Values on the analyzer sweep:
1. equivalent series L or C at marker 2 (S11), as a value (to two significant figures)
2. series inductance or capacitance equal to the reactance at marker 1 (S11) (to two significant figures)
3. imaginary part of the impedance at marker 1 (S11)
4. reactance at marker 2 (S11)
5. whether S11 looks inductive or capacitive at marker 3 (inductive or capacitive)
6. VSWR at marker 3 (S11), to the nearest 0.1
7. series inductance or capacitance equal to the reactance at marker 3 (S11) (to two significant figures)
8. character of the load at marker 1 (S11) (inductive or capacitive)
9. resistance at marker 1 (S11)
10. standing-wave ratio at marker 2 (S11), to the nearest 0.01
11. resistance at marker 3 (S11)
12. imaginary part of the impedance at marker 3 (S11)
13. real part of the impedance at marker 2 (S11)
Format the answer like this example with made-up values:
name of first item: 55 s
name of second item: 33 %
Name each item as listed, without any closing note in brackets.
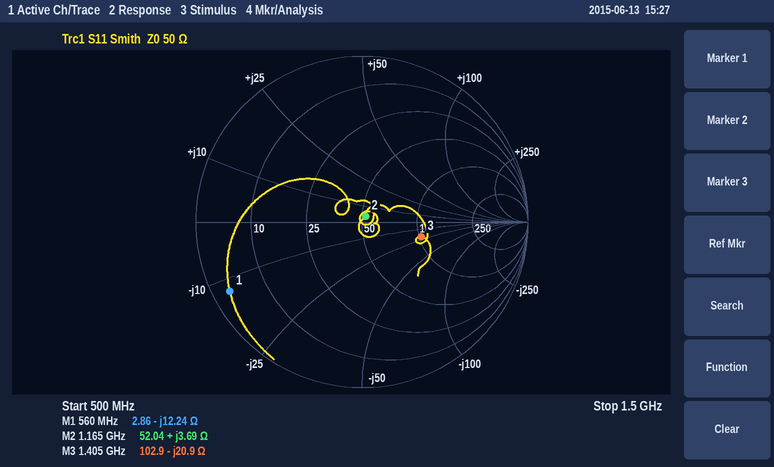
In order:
equivalent series L or C at marker 2 (S11), as a value: 500 pH
series inductance or capacitance equal to the reactance at marker 1 (S11): 23 pF
imaginary part of the impedance at marker 1: -12.24 Ω
reactance at marker 2: +3.69 Ω
whether S11 looks inductive or capacitive at marker 3: capacitive
VSWR at marker 3 (S11), to the nearest 0.1: 2.2
series inductance or capacitance equal to the reactance at marker 3 (S11): 5.4 pF
character of the load at marker 1 (S11): capacitive
resistance at marker 1: 2.86 Ω
standing-wave ratio at marker 2 (S11), to the nearest 0.01: 1.09
resistance at marker 3: 102.9 Ω
imaginary part of the impedance at marker 3: -20.9 Ω
real part of the impedance at marker 2: 52.04 Ω
